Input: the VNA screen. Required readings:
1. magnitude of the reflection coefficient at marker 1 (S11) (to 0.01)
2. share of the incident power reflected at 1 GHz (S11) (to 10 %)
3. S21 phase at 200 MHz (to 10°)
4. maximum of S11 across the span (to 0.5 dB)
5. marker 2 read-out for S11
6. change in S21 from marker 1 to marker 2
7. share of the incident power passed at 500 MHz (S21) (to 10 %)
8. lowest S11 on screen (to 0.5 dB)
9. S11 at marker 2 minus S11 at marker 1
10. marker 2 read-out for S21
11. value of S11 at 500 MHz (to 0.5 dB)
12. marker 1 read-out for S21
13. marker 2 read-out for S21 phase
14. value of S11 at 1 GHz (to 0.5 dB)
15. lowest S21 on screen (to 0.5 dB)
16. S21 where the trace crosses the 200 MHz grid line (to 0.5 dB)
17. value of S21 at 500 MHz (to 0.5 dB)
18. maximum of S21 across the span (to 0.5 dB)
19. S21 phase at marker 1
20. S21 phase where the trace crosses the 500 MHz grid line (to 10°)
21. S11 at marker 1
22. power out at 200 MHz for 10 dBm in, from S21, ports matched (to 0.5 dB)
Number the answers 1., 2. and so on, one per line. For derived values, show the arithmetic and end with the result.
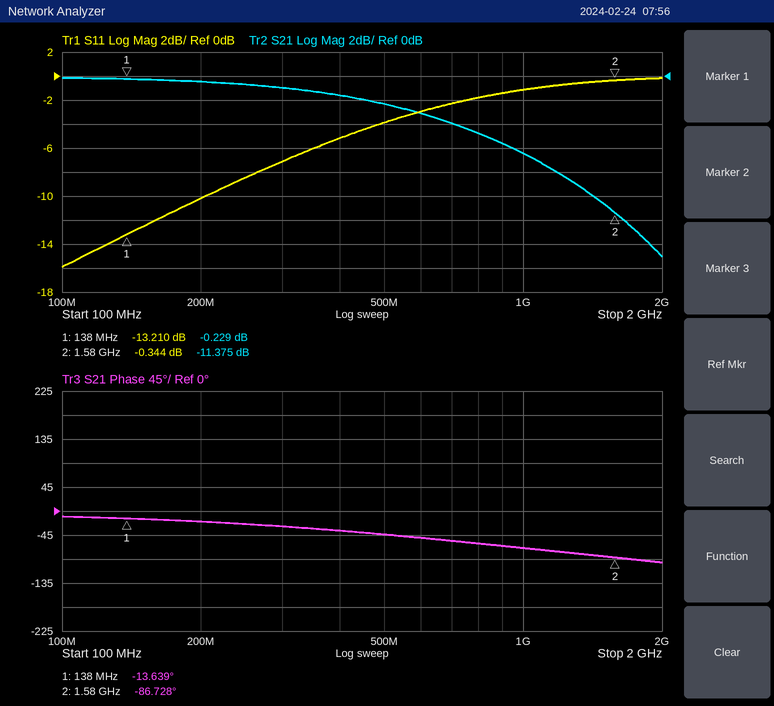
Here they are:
1. 10^(-13.21/20) ≈ 0.22
2. 10^(-1/10) ≈ 79.4 %, so 80 % to the nearest 10 %
3. -20°
4. 0.0 dB
5. -0.344 dB
6. -11.375 − (-0.229) = -11.146 dB
7. 10^(-2.5/10) ≈ 56.2 %, so 60 % to the nearest 10 %
8. -16.0 dB
9. -0.344 − (-13.21) = 12.866 dB
10. -11.375 dB
11. -4.0 dB
12. -0.229 dB
13. -86.728°
14. -1.0 dB
15. -15.0 dB
16. -0.5 dB
17. -2.5 dB
18. 0.0 dB
19. -13.639°
20. -40°
21. -13.210 dB
22. 10 dBm + (-0.5 dB) = 9.5 dBm
